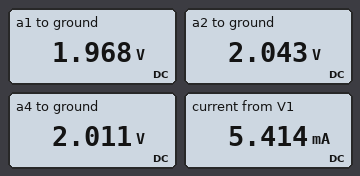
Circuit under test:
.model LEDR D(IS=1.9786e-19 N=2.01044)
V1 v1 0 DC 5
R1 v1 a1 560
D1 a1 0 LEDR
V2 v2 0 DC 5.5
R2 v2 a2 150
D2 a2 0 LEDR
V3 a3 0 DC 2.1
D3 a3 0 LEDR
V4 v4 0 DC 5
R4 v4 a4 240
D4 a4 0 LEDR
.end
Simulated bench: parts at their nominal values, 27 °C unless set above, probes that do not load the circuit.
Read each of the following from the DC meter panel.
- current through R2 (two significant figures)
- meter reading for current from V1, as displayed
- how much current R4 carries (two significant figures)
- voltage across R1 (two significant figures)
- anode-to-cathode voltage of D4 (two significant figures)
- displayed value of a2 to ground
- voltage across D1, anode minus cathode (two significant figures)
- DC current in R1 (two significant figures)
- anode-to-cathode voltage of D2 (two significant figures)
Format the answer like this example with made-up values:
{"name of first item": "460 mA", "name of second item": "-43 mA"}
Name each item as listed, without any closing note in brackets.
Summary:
{"current through R2": "23 mA", "meter reading for current from V1, as displayed": "5.414 mA", "how much current R4 carries": "12 mA", "voltage across R1": "3.0 V", "anode-to-cathode voltage of D4": "2.0 V", "displayed value of a2 to ground": "2.043 V", "voltage across D1, anode minus cathode": "2.0 V", "DC current in R1": "5.4 mA", "anode-to-cathode voltage of D2": "2.0 V"}
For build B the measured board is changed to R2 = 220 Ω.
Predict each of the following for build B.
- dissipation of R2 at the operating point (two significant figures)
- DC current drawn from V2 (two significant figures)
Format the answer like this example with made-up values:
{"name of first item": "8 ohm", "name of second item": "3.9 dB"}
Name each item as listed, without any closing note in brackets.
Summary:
{"dissipation of R2 at the operating point": "55 mW", "DC current drawn from V2": "16 mA"}
